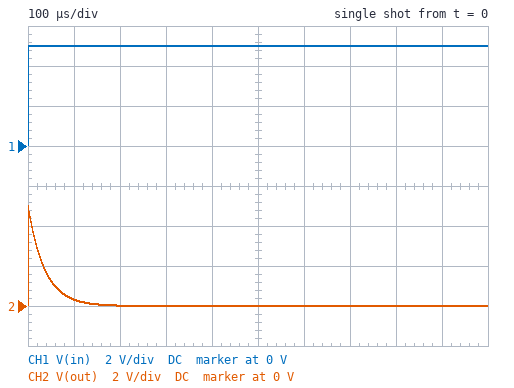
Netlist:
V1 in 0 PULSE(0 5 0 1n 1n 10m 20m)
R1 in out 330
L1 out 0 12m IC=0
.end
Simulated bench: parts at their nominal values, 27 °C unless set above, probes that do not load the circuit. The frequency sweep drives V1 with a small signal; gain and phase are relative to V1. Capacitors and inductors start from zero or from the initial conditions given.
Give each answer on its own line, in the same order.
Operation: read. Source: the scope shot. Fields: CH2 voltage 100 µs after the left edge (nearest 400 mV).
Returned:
400 mV
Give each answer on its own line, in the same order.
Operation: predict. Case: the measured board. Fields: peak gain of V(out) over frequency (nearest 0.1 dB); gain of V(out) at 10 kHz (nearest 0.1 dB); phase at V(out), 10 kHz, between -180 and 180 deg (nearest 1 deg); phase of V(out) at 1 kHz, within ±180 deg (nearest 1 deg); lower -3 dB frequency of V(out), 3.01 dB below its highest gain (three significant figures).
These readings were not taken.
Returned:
0 dB
-0.8 dB
24 deg
77 deg
4.38 kHz
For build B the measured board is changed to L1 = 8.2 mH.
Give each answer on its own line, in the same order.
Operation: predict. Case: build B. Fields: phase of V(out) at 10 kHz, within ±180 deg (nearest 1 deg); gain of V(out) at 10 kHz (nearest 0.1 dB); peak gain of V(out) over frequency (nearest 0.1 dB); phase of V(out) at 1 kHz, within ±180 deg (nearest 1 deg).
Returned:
33 deg
-1.5 dB
0 dB
81 deg
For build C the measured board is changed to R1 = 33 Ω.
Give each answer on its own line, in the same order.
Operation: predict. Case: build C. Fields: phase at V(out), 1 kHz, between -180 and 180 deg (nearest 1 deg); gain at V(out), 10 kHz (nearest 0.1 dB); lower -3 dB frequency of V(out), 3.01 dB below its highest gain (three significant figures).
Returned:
24 deg
0 dB
438 Hz
